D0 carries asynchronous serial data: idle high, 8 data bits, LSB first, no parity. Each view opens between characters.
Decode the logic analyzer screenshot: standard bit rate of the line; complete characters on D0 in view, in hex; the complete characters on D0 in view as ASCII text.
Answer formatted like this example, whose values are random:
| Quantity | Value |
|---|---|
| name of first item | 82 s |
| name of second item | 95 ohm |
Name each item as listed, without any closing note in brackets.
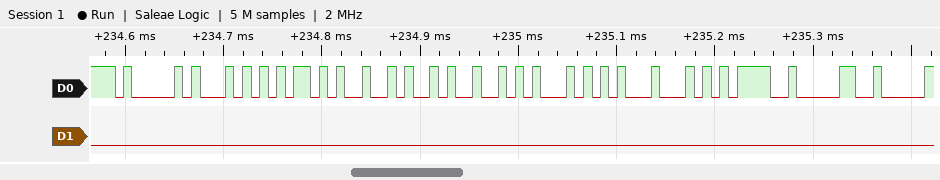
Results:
| Quantity | Value |
|---|---|
| standard bit rate of the line | 115200 baud |
| complete characters on D0 in view, in hex | 41, 54, 2B, 4A, 52, 54, 44, 3D, 30 |
| the complete characters on D0 in view as ASCII text | "AT+JRTD=0" |
